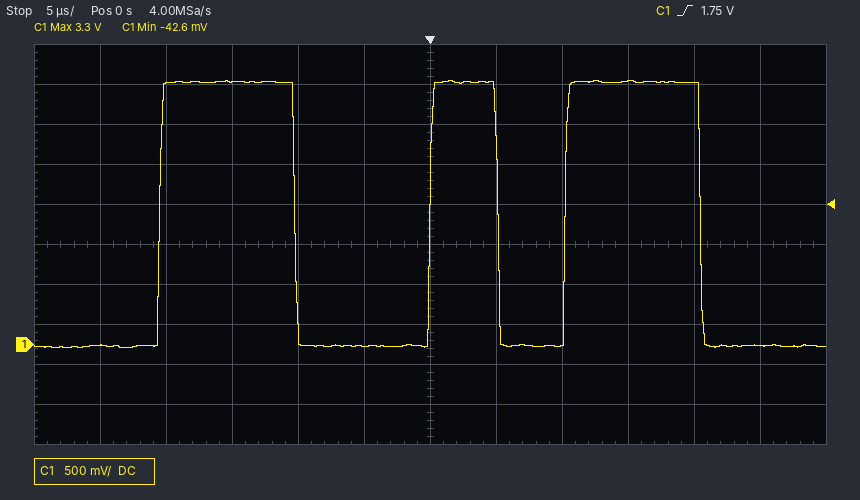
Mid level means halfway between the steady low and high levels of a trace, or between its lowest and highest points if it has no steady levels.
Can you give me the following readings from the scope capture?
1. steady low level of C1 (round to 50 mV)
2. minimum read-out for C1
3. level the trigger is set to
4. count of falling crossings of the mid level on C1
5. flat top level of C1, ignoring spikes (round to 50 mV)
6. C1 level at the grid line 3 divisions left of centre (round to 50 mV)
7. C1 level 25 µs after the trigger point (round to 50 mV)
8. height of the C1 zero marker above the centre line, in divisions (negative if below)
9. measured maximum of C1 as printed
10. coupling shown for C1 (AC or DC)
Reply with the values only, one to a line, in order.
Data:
0 mV
-42.6 mV
1.75 V
3
3.30 V
3.30 V
0 mV
-2.5 div
3.3 V
DC
